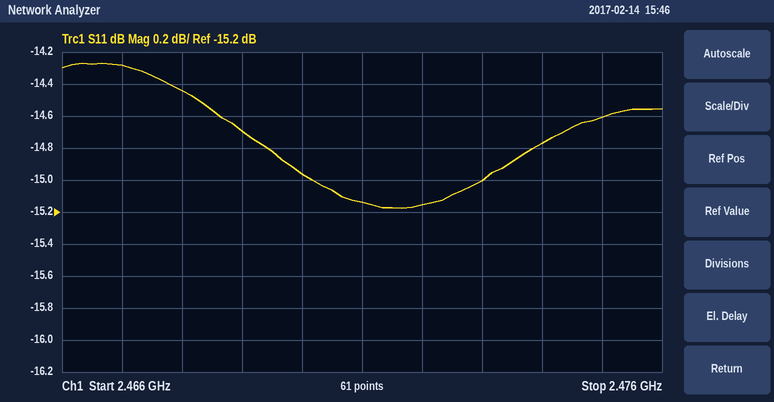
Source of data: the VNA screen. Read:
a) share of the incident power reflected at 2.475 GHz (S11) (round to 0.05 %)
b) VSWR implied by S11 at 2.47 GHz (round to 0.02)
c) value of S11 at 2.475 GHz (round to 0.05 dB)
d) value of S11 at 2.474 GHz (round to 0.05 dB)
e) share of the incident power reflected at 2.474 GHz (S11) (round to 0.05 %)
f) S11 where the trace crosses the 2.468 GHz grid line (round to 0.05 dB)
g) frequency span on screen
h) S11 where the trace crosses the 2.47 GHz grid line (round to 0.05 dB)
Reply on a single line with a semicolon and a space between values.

3.45 %; 1.44; -14.60 dB; -14.75 dB; 3.35 %; -14.45 dB; 10 MHz; -14.95 dB
